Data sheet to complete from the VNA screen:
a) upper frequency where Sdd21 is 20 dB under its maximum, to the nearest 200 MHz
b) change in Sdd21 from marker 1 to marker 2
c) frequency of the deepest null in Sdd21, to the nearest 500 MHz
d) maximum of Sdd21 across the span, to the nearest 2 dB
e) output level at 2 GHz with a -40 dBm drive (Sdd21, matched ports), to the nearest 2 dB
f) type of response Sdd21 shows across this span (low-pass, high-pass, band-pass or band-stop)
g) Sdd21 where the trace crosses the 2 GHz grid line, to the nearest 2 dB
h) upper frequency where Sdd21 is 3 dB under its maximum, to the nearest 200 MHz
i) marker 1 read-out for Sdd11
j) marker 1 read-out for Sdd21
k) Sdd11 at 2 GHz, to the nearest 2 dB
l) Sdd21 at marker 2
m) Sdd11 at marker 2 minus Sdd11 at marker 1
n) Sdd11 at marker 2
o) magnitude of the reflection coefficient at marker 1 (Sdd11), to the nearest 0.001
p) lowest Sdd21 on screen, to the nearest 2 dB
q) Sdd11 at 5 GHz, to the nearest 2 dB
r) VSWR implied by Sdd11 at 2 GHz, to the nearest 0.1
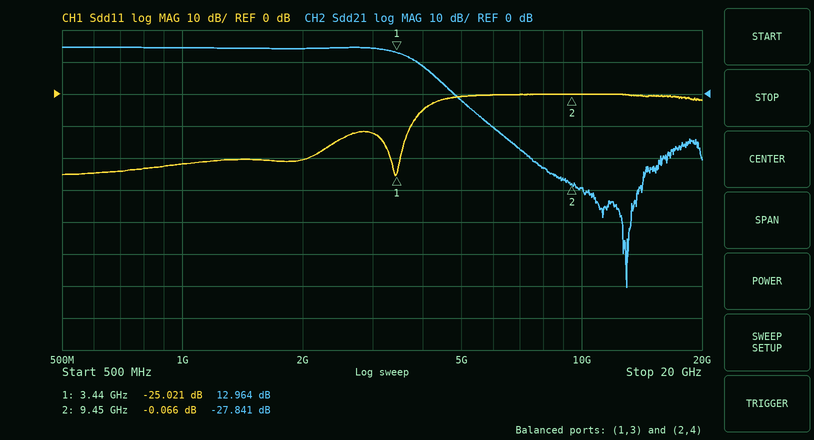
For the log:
5.4 GHz
-40.805 dB
13.0 GHz
14 dB
-26 dBm
low-pass
14 dB
3.6 GHz
-25.021 dB
12.964 dB
-20 dB
-27.841 dB
24.955 dB
-0.066 dB
0.056
-60 dB
0 dB
1.2
